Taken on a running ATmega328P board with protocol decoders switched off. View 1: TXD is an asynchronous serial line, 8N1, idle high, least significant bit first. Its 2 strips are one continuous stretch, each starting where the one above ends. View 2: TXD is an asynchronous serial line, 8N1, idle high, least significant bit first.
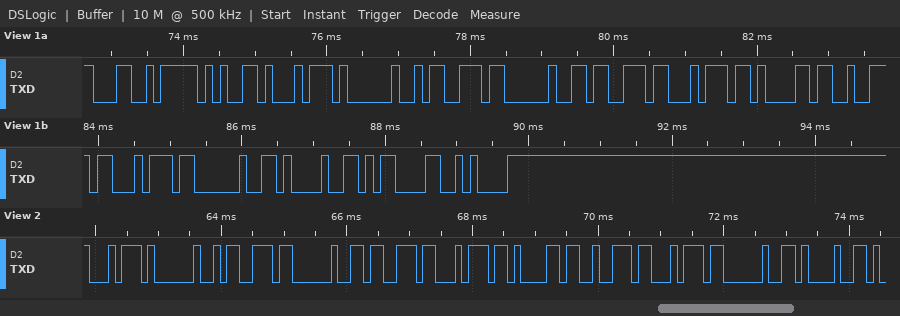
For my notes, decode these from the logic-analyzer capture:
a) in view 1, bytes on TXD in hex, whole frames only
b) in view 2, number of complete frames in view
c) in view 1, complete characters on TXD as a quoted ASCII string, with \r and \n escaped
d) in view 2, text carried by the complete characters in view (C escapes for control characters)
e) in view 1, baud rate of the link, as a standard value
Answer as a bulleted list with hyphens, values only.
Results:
- 0x4C 0x65 0x74 0x20 0x73 0x20 0x73 0x74 0x61 0x72 0x74 0x20 0x21 0x0D 0x0A
- 11
- "Let s start !\r\n"
- "t s start !"
- 9600 baud
